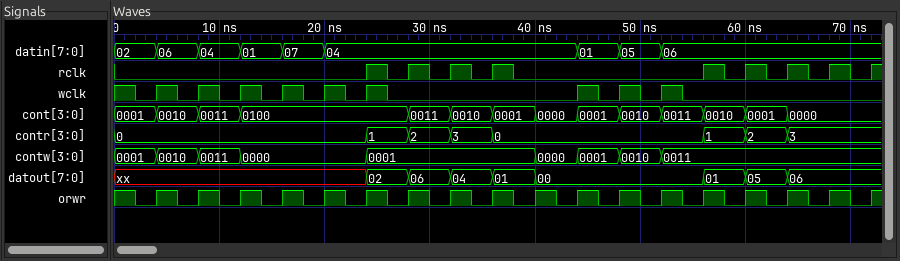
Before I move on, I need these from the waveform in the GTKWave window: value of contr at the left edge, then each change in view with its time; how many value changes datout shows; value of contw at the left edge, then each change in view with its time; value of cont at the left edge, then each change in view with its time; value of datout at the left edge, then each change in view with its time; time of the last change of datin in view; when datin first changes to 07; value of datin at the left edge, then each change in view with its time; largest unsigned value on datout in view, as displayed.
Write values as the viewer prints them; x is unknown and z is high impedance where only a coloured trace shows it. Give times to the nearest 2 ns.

0, 1 at 24 ns, 2 at 28 ns, 3 at 32 ns, 0 at 36 ns, 1 at 56 ns, 2 at 60 ns, 3 at 64 ns
8
0001, 0010 at 4 ns, 0011 at 8 ns, 0000 at 12 ns, 0001 at 24 ns, 0000 at 40 ns, 0001 at 44 ns, 0010 at 48 ns, 0011 at 52 ns
0001, 0010 at 4 ns, 0011 at 8 ns, 0100 at 12 ns, 0011 at 28 ns, 0010 at 32 ns, 0001 at 36 ns, 0000 at 40 ns, 0001 at 44 ns, 0010 at 48 ns, 0011 at 52 ns, 0010 at 56 ns, 0001 at 60 ns, 0000 at 64 ns
xx, 02 at 24 ns, 06 at 28 ns, 04 at 32 ns, 01 at 36 ns, 00 at 40 ns, 01 at 56 ns, 05 at 60 ns, 06 at 64 ns
52 ns
16 ns
02, 06 at 4 ns, 04 at 8 ns, 01 at 12 ns, 07 at 16 ns, 04 at 20 ns, 01 at 44 ns, 05 at 48 ns, 06 at 52 ns
06
